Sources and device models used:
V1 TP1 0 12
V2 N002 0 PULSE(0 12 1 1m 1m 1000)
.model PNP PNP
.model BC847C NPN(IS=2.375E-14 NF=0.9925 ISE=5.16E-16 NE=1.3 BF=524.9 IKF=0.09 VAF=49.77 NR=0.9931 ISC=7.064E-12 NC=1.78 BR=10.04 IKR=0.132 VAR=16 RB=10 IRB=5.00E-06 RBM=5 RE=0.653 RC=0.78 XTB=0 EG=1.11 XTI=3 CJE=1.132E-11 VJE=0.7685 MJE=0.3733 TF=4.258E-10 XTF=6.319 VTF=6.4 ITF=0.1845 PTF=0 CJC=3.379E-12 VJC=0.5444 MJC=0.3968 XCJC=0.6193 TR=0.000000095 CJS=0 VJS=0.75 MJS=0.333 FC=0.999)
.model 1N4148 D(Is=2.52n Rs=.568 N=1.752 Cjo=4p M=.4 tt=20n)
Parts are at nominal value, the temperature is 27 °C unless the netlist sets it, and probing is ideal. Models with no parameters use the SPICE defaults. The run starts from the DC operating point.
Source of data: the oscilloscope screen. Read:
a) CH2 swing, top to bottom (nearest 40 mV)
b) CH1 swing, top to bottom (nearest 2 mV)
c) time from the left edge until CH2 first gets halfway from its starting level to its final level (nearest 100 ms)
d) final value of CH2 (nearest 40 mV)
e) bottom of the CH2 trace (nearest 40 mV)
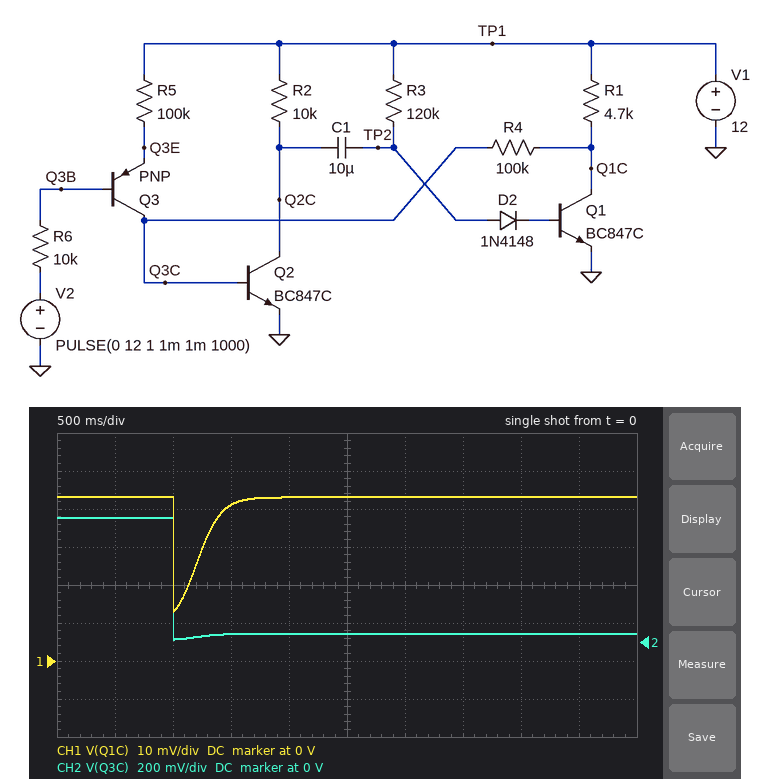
640 mV
30 mV
1.0 s
40 mV
0 V
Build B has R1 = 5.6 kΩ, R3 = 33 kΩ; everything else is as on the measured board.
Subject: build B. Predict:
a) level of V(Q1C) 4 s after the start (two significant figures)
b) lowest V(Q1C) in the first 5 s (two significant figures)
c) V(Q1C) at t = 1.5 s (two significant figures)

20 mV
11 mV
19 mV
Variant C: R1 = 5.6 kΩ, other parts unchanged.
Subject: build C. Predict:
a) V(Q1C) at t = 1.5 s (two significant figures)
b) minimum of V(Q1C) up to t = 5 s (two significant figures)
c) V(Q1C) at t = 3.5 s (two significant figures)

37 mV
11 mV
39 mV
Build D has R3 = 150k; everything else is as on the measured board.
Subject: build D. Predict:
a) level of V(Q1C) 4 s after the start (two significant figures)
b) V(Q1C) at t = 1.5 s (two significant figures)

48 mV
45 mV
